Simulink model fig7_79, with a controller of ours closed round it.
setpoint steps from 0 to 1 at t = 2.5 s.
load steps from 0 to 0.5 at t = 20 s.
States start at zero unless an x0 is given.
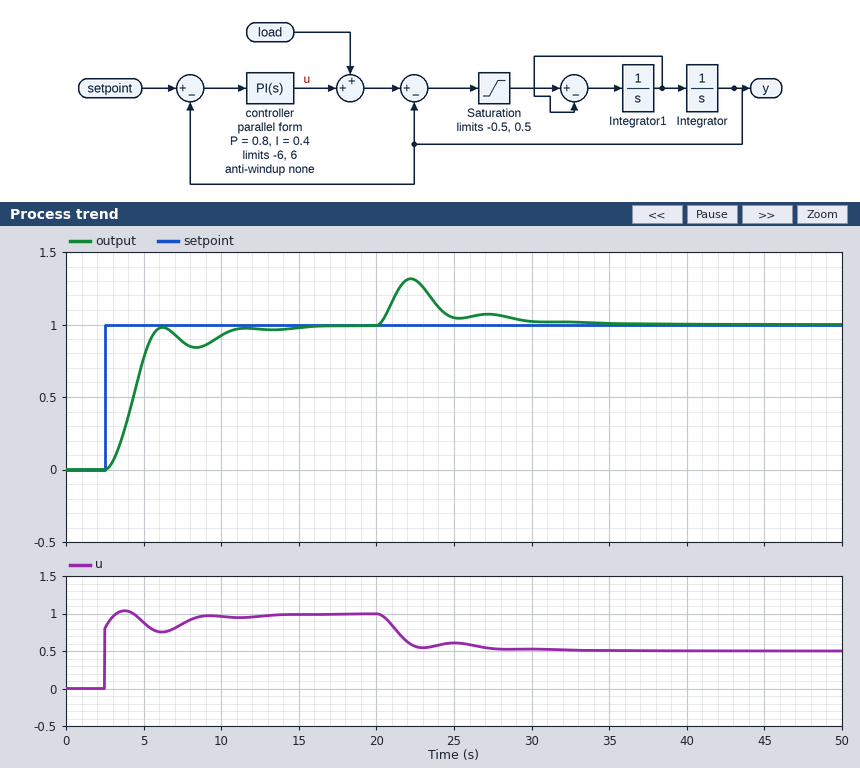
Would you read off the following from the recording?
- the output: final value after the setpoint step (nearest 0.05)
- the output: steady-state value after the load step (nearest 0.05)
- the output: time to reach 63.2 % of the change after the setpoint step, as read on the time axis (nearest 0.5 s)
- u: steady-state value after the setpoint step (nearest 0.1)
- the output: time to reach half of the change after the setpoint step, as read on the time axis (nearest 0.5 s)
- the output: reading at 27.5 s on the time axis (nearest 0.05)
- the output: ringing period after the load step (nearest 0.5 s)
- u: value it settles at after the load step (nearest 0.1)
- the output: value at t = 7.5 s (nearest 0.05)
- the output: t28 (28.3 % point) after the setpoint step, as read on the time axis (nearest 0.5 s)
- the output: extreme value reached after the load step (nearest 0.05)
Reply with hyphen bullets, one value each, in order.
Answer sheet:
- 1.00
- 1.00
- 4.5 s
- 1.0
- 4.5 s
- 1.05
- 5.0 s
- 0.5
- 0.90
- 4.0 s
- 1.30
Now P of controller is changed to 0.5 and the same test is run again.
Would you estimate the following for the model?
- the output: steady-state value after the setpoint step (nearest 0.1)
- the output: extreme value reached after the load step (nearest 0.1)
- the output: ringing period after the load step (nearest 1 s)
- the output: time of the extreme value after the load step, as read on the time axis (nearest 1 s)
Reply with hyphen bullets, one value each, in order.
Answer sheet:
- 1.0
- 1.4
- 6 s
- 22 s
